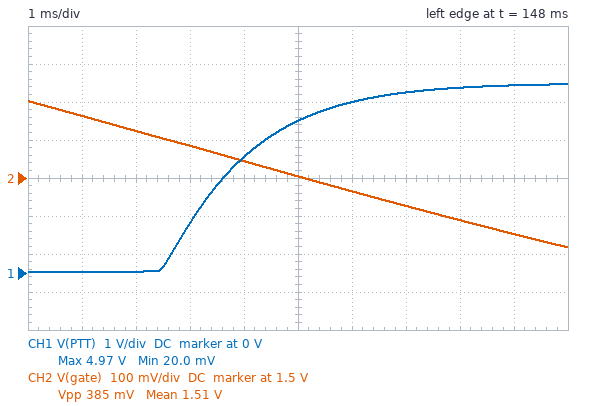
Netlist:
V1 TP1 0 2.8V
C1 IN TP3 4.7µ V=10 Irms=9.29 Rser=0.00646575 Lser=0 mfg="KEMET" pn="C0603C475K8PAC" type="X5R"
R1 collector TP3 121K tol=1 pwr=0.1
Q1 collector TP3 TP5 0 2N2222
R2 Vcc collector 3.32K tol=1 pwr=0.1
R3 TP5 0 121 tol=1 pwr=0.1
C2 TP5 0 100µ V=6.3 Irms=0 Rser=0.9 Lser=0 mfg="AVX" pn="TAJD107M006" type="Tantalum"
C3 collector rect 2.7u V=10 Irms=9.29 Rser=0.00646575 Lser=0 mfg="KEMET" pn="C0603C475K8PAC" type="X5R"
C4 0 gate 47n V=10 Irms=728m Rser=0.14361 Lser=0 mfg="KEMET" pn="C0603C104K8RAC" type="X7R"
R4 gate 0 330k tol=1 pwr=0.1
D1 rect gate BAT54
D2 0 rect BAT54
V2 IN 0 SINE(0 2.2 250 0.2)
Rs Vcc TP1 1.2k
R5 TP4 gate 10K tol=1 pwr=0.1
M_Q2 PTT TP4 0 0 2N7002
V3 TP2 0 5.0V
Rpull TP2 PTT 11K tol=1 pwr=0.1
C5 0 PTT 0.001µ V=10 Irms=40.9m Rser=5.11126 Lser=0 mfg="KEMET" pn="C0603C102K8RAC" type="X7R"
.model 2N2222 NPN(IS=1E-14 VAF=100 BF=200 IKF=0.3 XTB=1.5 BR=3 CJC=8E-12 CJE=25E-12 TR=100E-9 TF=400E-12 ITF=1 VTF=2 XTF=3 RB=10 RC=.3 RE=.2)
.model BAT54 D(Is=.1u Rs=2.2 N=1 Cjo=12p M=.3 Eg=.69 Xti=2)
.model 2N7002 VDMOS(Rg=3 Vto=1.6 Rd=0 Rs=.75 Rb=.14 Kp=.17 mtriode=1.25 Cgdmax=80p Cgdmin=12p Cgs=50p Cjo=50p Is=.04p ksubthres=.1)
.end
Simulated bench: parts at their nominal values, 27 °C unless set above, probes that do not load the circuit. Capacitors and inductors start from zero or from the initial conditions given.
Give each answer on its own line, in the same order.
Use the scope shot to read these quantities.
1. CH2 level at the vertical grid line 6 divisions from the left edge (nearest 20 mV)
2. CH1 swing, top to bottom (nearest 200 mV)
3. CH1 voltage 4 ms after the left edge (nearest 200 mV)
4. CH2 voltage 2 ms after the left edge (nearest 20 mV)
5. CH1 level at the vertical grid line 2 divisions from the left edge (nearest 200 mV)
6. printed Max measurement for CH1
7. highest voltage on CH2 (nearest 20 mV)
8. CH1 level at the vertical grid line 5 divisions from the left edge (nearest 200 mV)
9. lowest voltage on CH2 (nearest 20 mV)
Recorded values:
1.46 V
5.0 V
3.0 V
1.62 V
0 V
4.97 V
1.70 V
4.0 V
1.32 V
